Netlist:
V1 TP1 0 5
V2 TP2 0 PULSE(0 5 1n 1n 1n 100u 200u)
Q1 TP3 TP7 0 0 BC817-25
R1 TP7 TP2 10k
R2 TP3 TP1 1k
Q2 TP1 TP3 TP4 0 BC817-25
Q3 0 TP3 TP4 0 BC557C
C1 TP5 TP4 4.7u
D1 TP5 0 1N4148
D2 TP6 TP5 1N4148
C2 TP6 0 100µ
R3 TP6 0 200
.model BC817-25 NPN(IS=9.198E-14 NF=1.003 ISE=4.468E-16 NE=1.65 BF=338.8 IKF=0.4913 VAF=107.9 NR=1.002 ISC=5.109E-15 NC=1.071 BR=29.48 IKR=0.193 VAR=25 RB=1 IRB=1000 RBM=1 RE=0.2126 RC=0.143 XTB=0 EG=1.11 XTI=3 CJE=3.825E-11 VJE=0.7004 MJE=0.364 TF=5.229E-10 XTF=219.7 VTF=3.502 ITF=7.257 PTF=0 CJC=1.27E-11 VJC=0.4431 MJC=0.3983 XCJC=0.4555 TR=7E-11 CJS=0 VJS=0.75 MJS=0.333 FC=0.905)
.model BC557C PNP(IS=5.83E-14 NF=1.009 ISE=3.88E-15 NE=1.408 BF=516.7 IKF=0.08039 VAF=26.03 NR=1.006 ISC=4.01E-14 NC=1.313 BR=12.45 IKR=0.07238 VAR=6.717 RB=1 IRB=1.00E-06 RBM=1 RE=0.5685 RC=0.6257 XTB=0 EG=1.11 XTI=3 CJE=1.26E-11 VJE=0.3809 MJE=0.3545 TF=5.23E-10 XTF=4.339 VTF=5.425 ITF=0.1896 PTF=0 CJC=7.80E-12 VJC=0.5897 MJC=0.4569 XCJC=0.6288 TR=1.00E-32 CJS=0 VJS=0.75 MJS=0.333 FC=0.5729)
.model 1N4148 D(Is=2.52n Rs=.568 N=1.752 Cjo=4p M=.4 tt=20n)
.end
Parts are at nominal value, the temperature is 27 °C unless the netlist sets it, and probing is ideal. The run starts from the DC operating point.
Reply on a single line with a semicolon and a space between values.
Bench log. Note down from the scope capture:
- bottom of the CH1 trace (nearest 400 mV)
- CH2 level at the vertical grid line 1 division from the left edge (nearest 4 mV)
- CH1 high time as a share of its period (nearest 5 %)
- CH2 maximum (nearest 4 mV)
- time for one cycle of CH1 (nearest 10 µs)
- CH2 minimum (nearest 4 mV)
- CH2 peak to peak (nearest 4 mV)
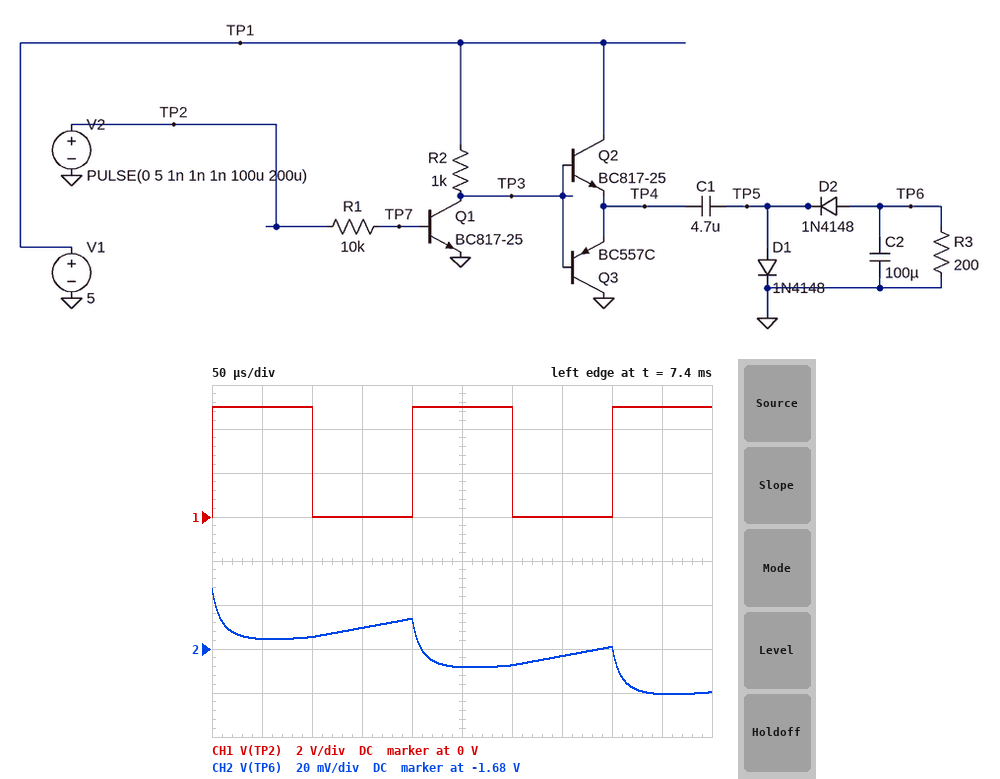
0 V; -1.676 V; 50 %; -1.652 V; 200 µs; -1.700 V; 48 mV
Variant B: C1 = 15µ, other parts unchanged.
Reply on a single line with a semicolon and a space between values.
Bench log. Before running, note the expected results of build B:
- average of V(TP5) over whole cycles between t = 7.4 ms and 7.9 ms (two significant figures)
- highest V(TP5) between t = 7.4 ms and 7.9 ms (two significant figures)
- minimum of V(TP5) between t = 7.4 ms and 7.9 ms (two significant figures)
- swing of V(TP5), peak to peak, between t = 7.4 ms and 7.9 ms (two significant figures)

-990 mV; 770 mV; -2.8 V; 3.5 V
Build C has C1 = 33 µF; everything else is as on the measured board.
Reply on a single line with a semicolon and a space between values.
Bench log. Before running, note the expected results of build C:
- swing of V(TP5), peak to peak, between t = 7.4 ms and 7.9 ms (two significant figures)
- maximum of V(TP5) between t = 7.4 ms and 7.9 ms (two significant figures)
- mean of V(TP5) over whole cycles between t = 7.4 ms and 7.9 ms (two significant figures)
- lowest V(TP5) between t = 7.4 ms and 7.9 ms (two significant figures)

3.5 V; 760 mV; -1.0 V; -2.8 V
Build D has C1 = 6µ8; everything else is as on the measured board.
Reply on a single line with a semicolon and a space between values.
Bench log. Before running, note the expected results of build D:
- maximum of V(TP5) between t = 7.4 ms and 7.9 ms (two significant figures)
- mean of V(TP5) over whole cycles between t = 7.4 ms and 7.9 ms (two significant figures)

820 mV; -920 mV
